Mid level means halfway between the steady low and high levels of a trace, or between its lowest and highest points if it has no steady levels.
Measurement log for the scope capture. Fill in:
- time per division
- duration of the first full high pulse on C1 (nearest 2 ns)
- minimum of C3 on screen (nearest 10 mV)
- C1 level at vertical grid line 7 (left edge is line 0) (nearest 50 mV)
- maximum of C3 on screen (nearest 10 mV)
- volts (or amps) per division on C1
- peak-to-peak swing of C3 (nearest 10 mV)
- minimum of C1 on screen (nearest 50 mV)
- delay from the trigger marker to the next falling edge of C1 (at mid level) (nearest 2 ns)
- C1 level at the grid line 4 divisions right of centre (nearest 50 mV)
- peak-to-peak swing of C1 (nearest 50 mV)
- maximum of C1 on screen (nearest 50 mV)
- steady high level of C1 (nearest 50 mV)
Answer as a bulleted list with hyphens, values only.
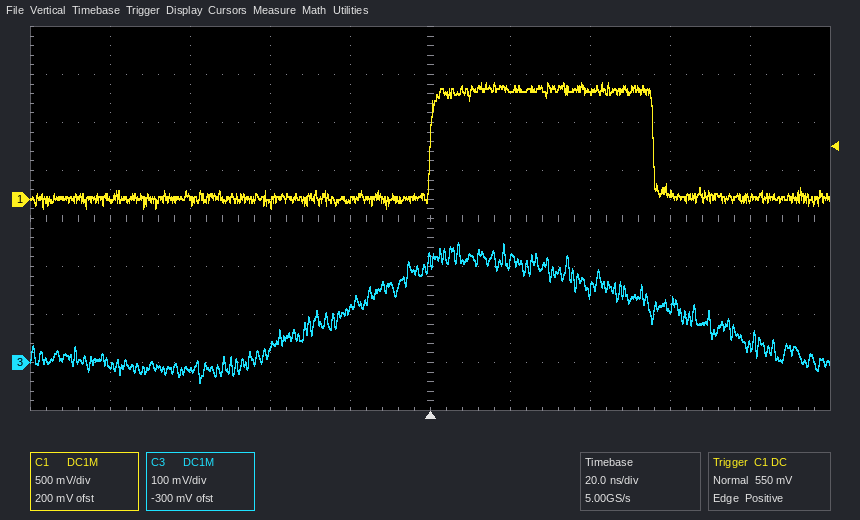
- 20 ns
- 56 ns
- -40 mV
- 1.10 V
- 250 mV
- 500 mV
- 290 mV
- -100 mV
- 56 ns
- 0 mV
- 1.30 V
- 1.20 V
- 1.15 V
